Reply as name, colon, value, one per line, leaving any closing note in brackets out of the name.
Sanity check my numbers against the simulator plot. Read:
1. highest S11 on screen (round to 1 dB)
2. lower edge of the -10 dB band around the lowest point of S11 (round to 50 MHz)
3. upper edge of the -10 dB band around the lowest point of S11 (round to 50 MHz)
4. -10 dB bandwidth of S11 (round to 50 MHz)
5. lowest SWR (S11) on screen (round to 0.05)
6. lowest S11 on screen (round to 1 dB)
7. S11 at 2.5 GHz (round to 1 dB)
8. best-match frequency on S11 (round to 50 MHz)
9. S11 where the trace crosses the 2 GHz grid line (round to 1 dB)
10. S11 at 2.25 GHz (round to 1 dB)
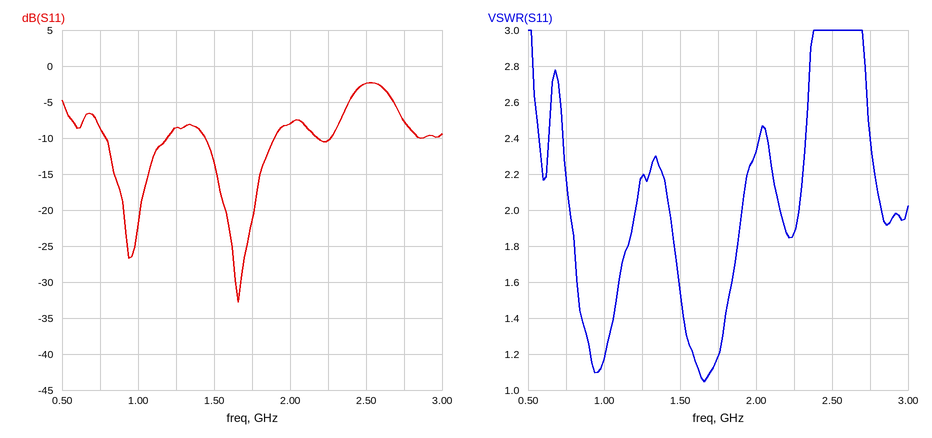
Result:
highest S11 on screen: -2 dB
lower edge of the -10 dB band around the lowest point of S11: 1.45 GHz
upper edge of the -10 dB band around the lowest point of S11: 1.90 GHz
-10 dB bandwidth of S11: 450 MHz
lowest SWR (S11) on screen: 1.05
lowest S11 on screen: -33 dB
S11 at 2.5 GHz: -2 dB
best-match frequency on S11: 1.65 GHz
S11 where the trace crosses the 2 GHz grid line: -8 dB
S11 at 2.25 GHz: -10 dB
